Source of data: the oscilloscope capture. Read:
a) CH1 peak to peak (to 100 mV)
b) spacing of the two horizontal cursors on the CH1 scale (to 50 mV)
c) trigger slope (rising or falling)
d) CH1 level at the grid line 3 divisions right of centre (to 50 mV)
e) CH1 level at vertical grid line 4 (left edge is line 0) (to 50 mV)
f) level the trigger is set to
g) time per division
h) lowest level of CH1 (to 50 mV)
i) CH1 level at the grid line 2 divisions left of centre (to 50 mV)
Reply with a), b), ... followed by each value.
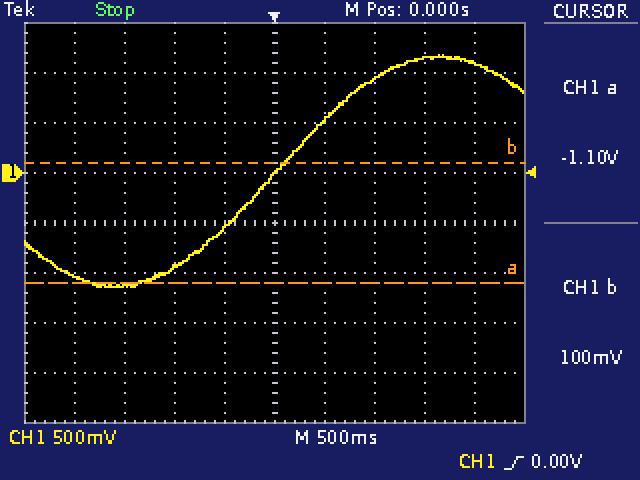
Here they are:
a) 2.30 V
b) 1.20 V
c) rising
d) 1.15 V
e) -550 mV
f) 0.00 V
g) 500 ms
h) -1.15 V
i) -950 mV
